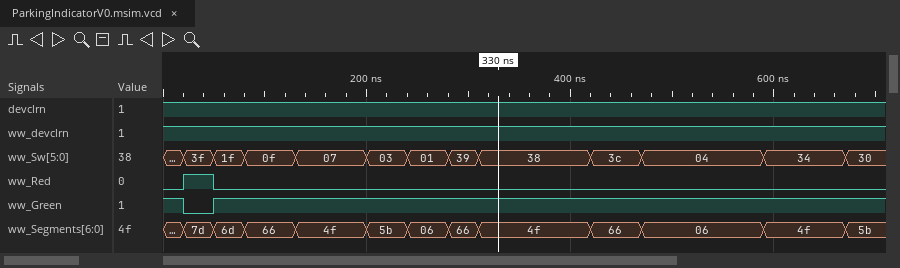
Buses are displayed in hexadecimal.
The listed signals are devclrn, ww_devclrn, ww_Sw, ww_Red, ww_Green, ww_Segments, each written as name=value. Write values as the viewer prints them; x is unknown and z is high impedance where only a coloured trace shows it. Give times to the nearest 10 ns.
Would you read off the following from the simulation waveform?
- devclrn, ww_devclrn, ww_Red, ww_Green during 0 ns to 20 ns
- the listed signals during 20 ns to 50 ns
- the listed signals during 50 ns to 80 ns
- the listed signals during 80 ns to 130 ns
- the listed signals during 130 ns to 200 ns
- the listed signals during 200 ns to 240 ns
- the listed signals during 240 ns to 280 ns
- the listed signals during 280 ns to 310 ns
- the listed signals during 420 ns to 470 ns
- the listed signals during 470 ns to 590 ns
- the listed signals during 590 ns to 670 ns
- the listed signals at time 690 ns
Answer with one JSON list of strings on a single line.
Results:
["devclrn=1, ww_devclrn=1, ww_Red=0, ww_Green=1", "devclrn=1, ww_devclrn=1, ww_Sw=3f, ww_Red=1, ww_Green=0, ww_Segments=7d", "devclrn=1, ww_devclrn=1, ww_Sw=1f, ww_Red=0, ww_Green=1, ww_Segments=6d", "devclrn=1, ww_devclrn=1, ww_Sw=0f, ww_Red=0, ww_Green=1, ww_Segments=66", "devclrn=1, ww_devclrn=1, ww_Sw=07, ww_Red=0, ww_Green=1, ww_Segments=4f", "devclrn=1, ww_devclrn=1, ww_Sw=03, ww_Red=0, ww_Green=1, ww_Segments=5b", "devclrn=1, ww_devclrn=1, ww_Sw=01, ww_Red=0, ww_Green=1, ww_Segments=06", "devclrn=1, ww_devclrn=1, ww_Sw=39, ww_Red=0, ww_Green=1, ww_Segments=66", "devclrn=1, ww_devclrn=1, ww_Sw=3c, ww_Red=0, ww_Green=1, ww_Segments=66", "devclrn=1, ww_devclrn=1, ww_Sw=04, ww_Red=0, ww_Green=1, ww_Segments=06", "devclrn=1, ww_devclrn=1, ww_Sw=34, ww_Red=0, ww_Green=1, ww_Segments=4f", "devclrn=1, ww_devclrn=1, ww_Sw=30, ww_Red=0, ww_Green=1, ww_Segments=5b"]
